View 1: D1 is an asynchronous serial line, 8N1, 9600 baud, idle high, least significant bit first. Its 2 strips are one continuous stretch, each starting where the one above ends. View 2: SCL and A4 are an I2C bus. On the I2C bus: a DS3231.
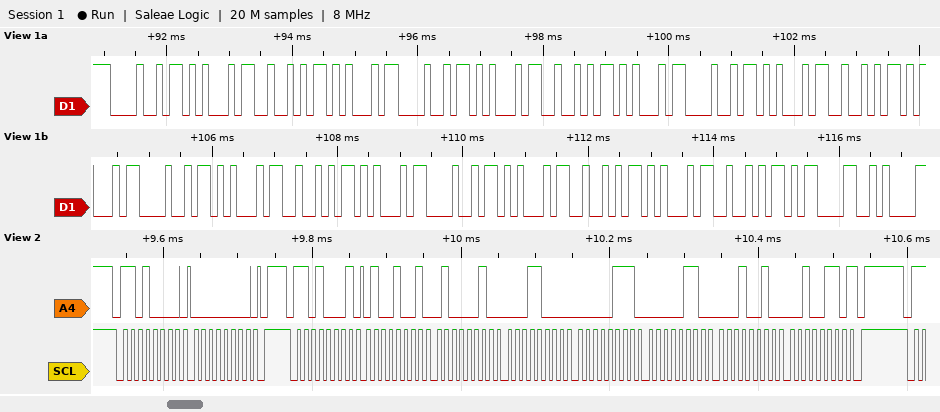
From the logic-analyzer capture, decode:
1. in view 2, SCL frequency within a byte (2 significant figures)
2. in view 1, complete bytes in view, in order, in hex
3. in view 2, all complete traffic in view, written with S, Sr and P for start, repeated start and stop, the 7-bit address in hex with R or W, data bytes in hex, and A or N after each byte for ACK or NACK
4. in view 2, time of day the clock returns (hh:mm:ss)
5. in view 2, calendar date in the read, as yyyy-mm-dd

100 kHz
48 45 52 45 48 45 52 45 48 45 52 45 48 45 52 45 48 45 52 45 52 0D 0A
S 68W A 00 A P S 68R A 49 A 42 A 18 A 07 A 06 A 12 A 26 N P
18:42:49
2026-12-06
